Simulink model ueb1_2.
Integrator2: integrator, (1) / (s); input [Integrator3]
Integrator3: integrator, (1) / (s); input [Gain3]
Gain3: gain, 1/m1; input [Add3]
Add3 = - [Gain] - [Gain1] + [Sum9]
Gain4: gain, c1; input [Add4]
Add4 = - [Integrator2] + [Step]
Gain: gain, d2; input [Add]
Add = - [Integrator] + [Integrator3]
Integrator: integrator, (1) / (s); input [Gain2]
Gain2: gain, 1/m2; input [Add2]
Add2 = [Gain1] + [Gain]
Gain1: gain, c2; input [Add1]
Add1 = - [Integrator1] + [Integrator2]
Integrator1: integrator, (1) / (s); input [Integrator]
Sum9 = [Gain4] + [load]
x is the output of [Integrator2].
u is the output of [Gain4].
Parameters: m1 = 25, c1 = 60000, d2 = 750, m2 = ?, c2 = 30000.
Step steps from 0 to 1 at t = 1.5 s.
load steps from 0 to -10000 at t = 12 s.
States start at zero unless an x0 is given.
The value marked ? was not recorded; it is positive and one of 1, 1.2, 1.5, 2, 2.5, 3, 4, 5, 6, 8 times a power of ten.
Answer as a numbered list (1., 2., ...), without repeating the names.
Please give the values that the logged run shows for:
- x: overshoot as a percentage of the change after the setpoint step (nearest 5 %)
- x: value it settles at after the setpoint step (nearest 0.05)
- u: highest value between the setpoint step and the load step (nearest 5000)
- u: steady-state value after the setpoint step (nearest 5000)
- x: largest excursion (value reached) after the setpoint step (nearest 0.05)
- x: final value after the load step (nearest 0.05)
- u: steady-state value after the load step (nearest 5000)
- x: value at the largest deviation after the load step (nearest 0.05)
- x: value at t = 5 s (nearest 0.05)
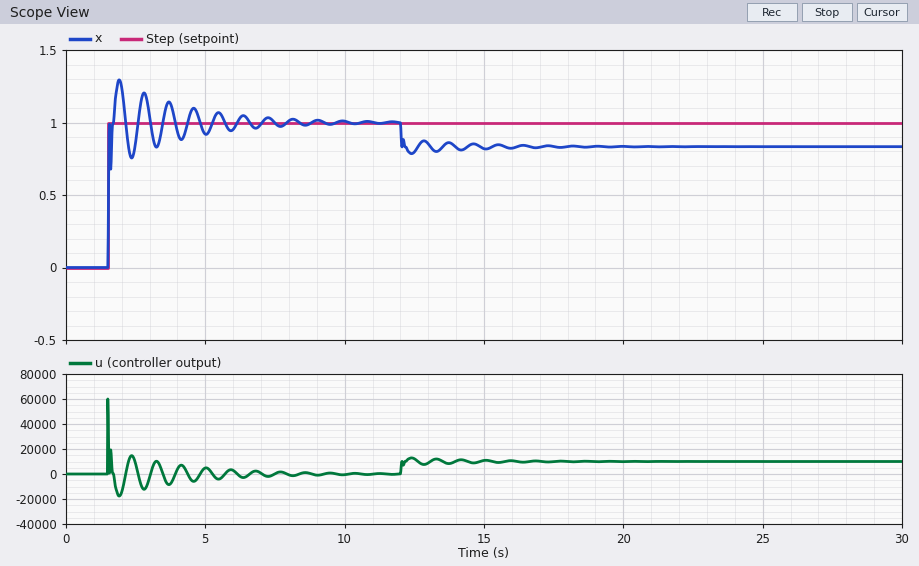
1. 30 %
2. 1.00
3. 60000
4. 0
5. 1.30
6. 0.85
7. 10000
8. 0.80
9. 0.90
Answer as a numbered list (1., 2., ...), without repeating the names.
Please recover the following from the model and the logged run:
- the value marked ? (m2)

1. 400
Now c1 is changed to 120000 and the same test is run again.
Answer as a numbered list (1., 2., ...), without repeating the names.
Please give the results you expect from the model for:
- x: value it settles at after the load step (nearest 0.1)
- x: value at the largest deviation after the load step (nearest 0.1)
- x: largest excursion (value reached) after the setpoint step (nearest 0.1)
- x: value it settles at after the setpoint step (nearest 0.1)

1. 0.9
2. 0.9
3. 1.2
4. 1.0
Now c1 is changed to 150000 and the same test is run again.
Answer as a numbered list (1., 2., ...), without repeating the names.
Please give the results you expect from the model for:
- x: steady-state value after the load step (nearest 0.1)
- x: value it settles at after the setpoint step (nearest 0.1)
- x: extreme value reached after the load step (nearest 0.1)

1. 0.9
2. 1.0
3. 0.9
